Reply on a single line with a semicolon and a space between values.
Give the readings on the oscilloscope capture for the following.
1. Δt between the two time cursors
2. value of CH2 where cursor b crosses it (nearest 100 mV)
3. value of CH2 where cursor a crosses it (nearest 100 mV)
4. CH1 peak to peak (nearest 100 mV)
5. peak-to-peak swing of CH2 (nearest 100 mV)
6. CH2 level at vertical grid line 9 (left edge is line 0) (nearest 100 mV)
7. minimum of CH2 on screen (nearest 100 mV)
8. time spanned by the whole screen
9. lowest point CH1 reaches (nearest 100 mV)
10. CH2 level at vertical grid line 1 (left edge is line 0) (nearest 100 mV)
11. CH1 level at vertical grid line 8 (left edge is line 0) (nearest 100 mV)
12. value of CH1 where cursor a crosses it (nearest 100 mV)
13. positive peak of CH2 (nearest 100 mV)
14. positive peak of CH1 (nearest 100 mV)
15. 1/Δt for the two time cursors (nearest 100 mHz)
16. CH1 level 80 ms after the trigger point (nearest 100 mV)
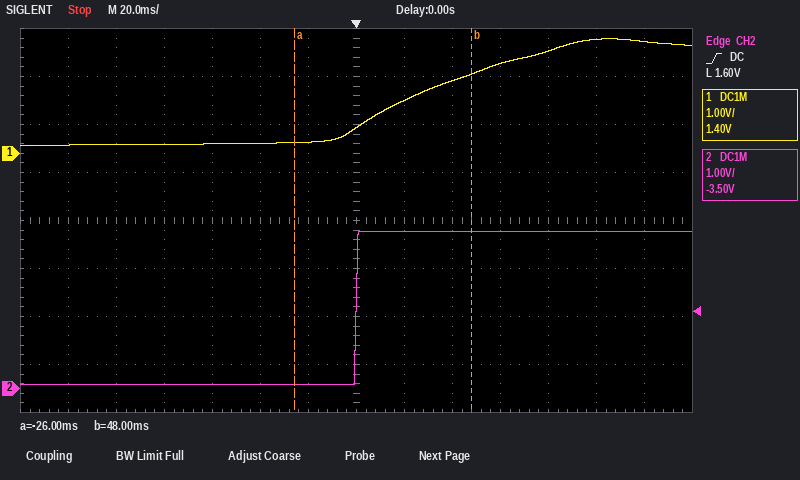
74 ms; 3.3 V; 100 mV; 2.2 V; 3.2 V; 3.3 V; 100 mV; 280 ms; 200 mV; 100 mV; 1.1 V; 200 mV; 3.3 V; 2.4 V; 13.5 Hz; 2.1 V
